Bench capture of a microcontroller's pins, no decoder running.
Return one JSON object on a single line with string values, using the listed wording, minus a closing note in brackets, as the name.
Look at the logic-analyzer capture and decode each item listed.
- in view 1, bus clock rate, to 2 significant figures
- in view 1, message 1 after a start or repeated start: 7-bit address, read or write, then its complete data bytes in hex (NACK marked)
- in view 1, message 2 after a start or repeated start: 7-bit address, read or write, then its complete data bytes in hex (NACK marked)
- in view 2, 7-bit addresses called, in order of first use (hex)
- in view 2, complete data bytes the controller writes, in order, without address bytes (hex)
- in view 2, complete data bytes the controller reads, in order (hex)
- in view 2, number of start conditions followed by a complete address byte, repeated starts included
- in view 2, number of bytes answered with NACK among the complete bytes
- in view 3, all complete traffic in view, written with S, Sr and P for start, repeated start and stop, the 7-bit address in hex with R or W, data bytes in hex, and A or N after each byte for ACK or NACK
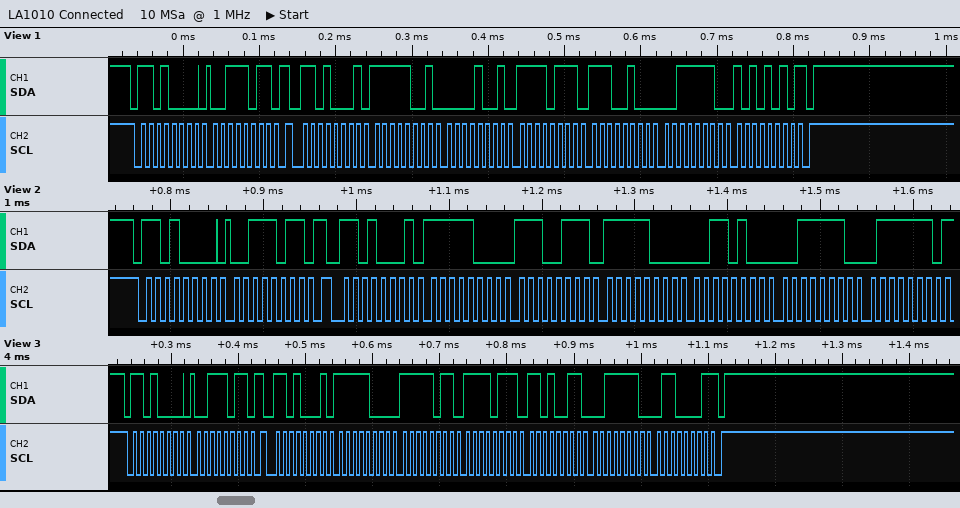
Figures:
{"in view 1, bus clock rate, to 2 significant figures": "100 kHz", "in view 1, message 1 after a start or repeated start: 7-bit address, read or write, then its complete data bytes in hex": "0x68 write: 3B", "in view 1, message 2 after a start or repeated start: 7-bit address, read or write, then its complete data bytes in hex": "0x68 read: F9 09 F7 E4 3E AA NACK", "in view 2, 7-bit addresses called, in order of first use": "0x68", "in view 2, complete data bytes the controller writes, in order, without address bytes": "3B", "in view 2, complete data bytes the controller reads, in order": "F8 E7 F8 34 3E 7E", "in view 2, number of start conditions followed by a complete address byte, repeated starts included": "2", "in view 2, number of bytes answered with NACK among the complete bytes": "1", "in view 3, all complete traffic in view, written with S, Sr and P for start, repeated start and stop, the 7-bit address in hex with R or W, data bytes in hex, and A or N after each byte for ACK or NACK": "S 68W A 3B A Sr 68R A F8 A FB A F7 A D3 A 3E A 61 N P"}
